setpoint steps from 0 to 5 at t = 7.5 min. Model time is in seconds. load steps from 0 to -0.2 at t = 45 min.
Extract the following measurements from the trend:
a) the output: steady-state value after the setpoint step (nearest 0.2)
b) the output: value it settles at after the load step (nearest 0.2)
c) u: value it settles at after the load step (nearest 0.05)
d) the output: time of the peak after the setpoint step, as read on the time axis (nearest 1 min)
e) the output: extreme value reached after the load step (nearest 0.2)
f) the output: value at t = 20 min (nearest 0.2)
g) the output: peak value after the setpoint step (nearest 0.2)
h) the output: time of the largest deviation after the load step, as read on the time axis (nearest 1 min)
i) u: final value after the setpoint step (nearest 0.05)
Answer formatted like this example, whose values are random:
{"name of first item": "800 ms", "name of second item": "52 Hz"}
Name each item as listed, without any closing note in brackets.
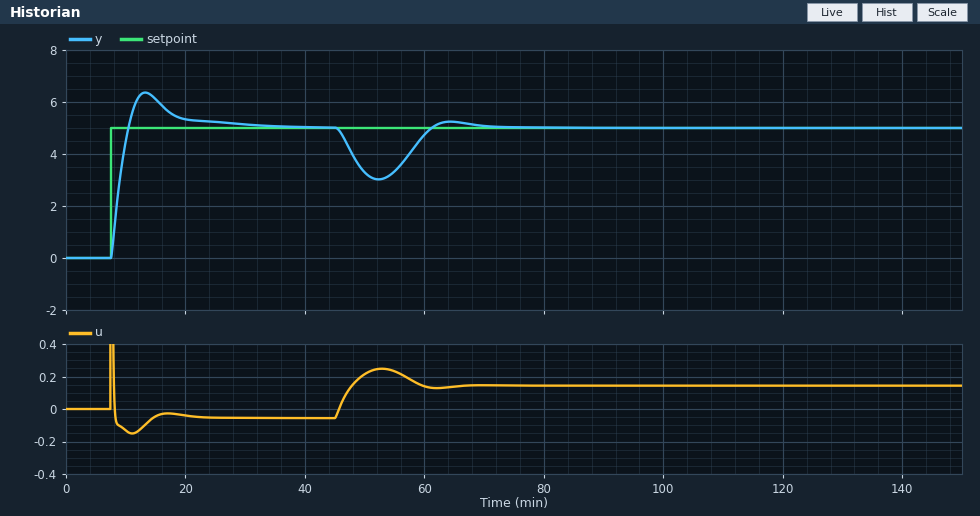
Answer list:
{"the output: steady-state value after the setpoint step": "5.0", "the output: value it settles at after the load step": "5.0", "u: value it settles at after the load step": "0.15", "the output: time of the peak after the setpoint step, as read on the time axis": "13 min", "the output: extreme value reached after the load step": "3.0", "the output: value at t = 20 min": "5.4", "the output: peak value after the setpoint step": "6.4", "the output: time of the largest deviation after the load step, as read on the time axis": "52 min", "u: final value after the setpoint step": "-0.05"}
